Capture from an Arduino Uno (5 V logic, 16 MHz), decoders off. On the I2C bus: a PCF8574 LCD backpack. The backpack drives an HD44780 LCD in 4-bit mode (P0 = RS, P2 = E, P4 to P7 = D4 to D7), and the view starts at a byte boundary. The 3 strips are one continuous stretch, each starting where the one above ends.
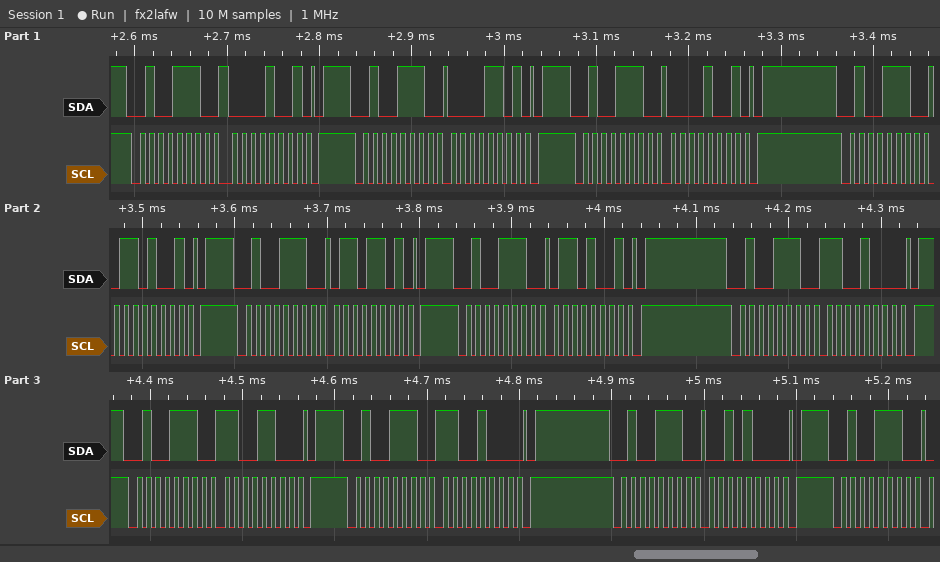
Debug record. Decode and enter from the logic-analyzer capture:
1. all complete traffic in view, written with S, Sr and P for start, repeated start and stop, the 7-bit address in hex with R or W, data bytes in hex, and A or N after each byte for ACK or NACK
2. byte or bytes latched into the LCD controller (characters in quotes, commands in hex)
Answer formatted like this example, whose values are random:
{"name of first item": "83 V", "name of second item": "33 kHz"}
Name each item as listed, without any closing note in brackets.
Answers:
{"all complete traffic in view, written with S, Sr and P for start, repeated start and stop, the 7-bit address in hex with R or W, data bytes in hex, and A or N after each byte for ACK or NACK": "S 27W A 09 A P S 27W A 0D A P S 27W A 09 A P S 27W A 69 A P S 27W A 6D A P S 27W A 69 A P S 27W A C8 A P S 27W A CC A P S 27W A C8 A P S 27W A 28 A P S 27W A", "byte or bytes latched into the LCD controller": "data 0x06"}
